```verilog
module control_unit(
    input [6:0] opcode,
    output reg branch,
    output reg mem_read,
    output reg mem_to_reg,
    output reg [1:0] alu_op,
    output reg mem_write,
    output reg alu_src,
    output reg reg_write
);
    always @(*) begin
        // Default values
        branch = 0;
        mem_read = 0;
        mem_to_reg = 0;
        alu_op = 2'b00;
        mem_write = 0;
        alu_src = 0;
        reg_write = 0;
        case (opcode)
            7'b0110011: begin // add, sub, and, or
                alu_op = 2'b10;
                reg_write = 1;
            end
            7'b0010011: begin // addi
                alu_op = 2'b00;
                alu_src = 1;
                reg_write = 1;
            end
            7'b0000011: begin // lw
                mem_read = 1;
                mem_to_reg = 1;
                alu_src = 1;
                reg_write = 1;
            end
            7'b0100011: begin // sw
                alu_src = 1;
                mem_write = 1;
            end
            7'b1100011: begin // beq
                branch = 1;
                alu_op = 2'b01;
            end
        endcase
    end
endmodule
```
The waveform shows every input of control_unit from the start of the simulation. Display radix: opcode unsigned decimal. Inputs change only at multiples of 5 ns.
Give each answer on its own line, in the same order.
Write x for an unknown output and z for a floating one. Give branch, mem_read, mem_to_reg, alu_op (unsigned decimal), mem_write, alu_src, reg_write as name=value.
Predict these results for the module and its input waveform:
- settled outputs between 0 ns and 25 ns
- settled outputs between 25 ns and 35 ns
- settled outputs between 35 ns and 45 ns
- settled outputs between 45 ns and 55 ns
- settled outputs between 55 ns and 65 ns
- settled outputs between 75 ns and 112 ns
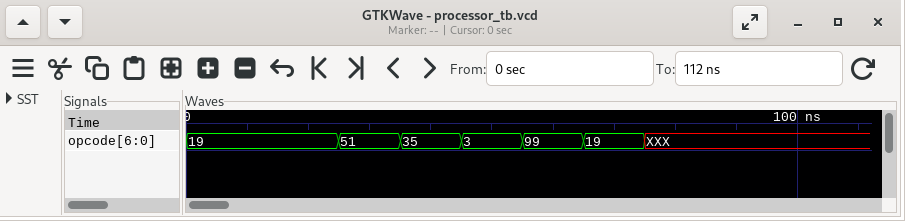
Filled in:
branch=0, mem_read=0, mem_to_reg=0, alu_op=0, mem_write=0, alu_src=1, reg_write=1
branch=0, mem_read=0, mem_to_reg=0, alu_op=2, mem_write=0, alu_src=0, reg_write=1
branch=0, mem_read=0, mem_to_reg=0, alu_op=0, mem_write=1, alu_src=1, reg_write=0
branch=0, mem_read=1, mem_to_reg=1, alu_op=0, mem_write=0, alu_src=1, reg_write=1
branch=1, mem_read=0, mem_to_reg=0, alu_op=1, mem_write=0, alu_src=0, reg_write=0
branch=0, mem_read=0, mem_to_reg=0, alu_op=0, mem_write=0, alu_src=0, reg_write=0
